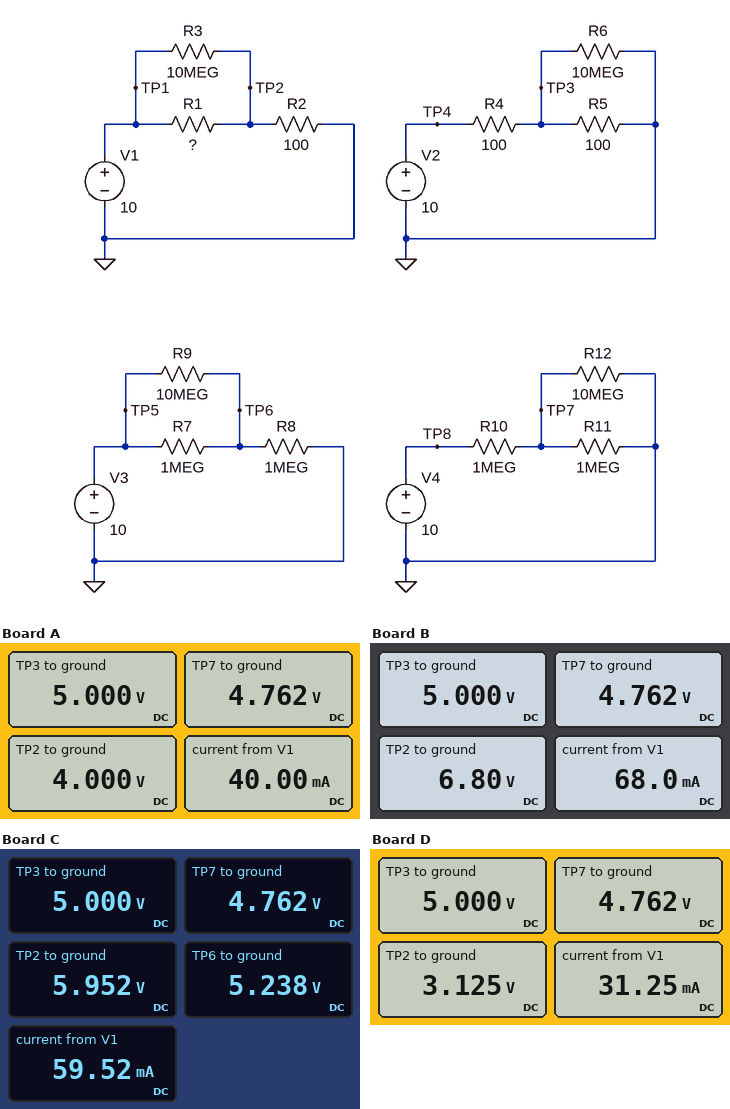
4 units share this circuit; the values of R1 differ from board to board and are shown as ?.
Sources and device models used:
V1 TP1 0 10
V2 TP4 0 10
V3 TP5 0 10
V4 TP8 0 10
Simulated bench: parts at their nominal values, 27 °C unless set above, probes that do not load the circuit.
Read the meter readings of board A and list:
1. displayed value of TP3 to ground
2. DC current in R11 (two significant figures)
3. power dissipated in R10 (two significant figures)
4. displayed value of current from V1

5.000 V
4.8 µA
27 µW
40.00 mA
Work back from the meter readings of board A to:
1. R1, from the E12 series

150 Ω
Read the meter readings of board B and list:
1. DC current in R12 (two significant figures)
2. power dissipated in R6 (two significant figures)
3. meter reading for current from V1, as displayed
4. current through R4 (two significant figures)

480 nA
2.5 µW
68.0 mA
50 mA
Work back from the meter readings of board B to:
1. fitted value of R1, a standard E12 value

47 Ω
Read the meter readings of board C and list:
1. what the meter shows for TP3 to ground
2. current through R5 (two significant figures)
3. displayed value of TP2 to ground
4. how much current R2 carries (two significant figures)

5.000 V
50 mA
5.952 V
60 mA
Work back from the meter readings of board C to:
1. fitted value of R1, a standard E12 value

68 Ω
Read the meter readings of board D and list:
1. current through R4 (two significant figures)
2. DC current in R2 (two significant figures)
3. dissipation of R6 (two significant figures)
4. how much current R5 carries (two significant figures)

50 mA
31 mA
2.5 µW
50 mA
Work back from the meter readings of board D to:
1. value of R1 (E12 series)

220 Ω
